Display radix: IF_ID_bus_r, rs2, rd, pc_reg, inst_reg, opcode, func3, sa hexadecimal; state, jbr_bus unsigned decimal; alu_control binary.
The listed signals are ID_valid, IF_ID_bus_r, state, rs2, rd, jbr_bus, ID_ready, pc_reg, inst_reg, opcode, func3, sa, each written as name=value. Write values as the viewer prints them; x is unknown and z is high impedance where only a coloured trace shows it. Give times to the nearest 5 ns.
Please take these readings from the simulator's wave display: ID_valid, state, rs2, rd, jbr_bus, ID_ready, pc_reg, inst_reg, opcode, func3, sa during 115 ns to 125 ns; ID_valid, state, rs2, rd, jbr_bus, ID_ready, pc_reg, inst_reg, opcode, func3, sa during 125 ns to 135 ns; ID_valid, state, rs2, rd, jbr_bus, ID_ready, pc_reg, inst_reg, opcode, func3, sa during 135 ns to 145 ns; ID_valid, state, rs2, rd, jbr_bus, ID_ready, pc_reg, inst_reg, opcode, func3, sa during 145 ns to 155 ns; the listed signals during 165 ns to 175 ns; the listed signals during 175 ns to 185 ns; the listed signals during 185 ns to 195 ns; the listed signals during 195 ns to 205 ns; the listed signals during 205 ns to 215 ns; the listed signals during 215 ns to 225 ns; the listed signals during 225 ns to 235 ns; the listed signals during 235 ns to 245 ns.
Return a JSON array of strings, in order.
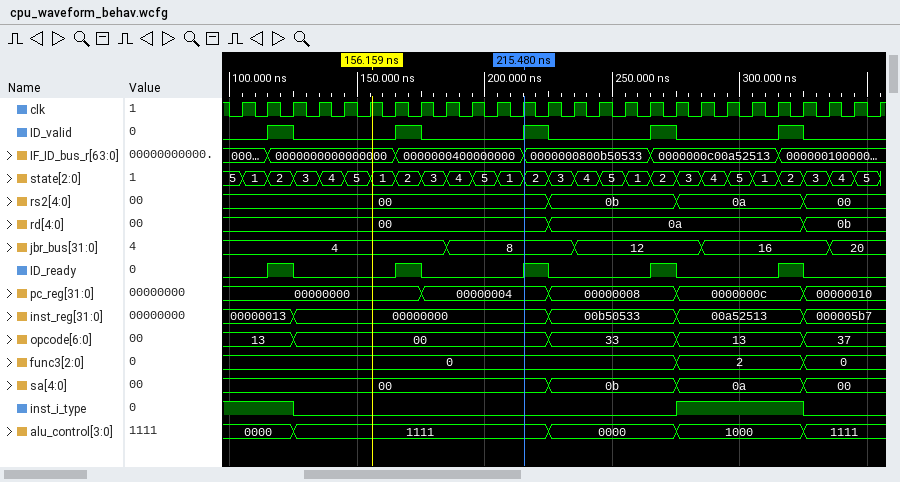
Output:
["ID_valid=1, state=2, rs2=00, rd=00, jbr_bus=4, ID_ready=1, pc_reg=00000000, inst_reg=00000013, opcode=13, func3=0, sa=00", "ID_valid=0, state=3, rs2=00, rd=00, jbr_bus=4, ID_ready=0, pc_reg=00000000, inst_reg=00000000, opcode=00, func3=0, sa=00", "ID_valid=0, state=4, rs2=00, rd=00, jbr_bus=4, ID_ready=0, pc_reg=00000000, inst_reg=00000000, opcode=00, func3=0, sa=00", "ID_valid=0, state=5, rs2=00, rd=00, jbr_bus=4, ID_ready=0, pc_reg=00000000, inst_reg=00000000, opcode=00, func3=0, sa=00", "ID_valid=1, IF_ID_bus_r=0000000400000000, state=2, rs2=00, rd=00, jbr_bus=4, ID_ready=1, pc_reg=00000000, inst_reg=00000000, opcode=00, func3=0, sa=00", "ID_valid=0, IF_ID_bus_r=0000000400000000, state=3, rs2=00, rd=00, jbr_bus=4, ID_ready=0, pc_reg=00000004, inst_reg=00000000, opcode=00, func3=0, sa=00", "ID_valid=0, IF_ID_bus_r=0000000400000000, state=4, rs2=00, rd=00, jbr_bus=8, ID_ready=0, pc_reg=00000004, inst_reg=00000000, opcode=00, func3=0, sa=00", "ID_valid=0, IF_ID_bus_r=0000000400000000, state=5, rs2=00, rd=00, jbr_bus=8, ID_ready=0, pc_reg=00000004, inst_reg=00000000, opcode=00, func3=0, sa=00", "ID_valid=0, IF_ID_bus_r=0000000400000000, state=1, rs2=00, rd=00, jbr_bus=8, ID_ready=0, pc_reg=00000004, inst_reg=00000000, opcode=00, func3=0, sa=00", "ID_valid=1, IF_ID_bus_r=0000000800b50533, state=2, rs2=00, rd=00, jbr_bus=8, ID_ready=1, pc_reg=00000004, inst_reg=00000000, opcode=00, func3=0, sa=00", "ID_valid=0, IF_ID_bus_r=0000000800b50533, state=3, rs2=0b, rd=0a, jbr_bus=8, ID_ready=0, pc_reg=00000008, inst_reg=00b50533, opcode=33, func3=0, sa=0b", "ID_valid=0, IF_ID_bus_r=0000000800b50533, state=4, rs2=0b, rd=0a, jbr_bus=12, ID_ready=0, pc_reg=00000008, inst_reg=00b50533, opcode=33, func3=0, sa=0b"]
